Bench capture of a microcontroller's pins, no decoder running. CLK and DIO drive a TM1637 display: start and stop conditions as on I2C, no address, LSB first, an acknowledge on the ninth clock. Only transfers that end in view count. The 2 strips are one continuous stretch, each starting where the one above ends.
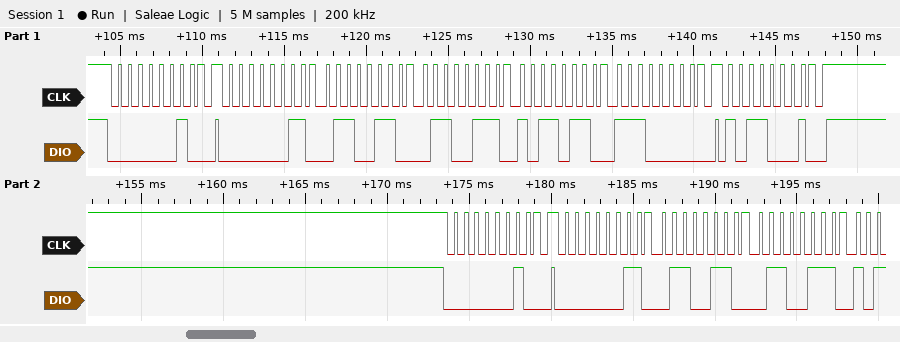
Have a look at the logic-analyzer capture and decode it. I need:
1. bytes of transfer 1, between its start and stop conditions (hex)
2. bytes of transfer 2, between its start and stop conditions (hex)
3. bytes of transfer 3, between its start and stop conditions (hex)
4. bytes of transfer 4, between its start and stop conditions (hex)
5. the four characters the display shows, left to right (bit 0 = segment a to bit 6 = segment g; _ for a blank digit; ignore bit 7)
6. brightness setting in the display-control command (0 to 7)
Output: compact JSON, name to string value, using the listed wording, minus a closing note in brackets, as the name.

{"bytes of transfer 1, between its start and stop conditions": "40", "bytes of transfer 2, between its start and stop conditions": "C0 66 E6 6D 07", "bytes of transfer 3, between its start and stop conditions": "8D", "bytes of transfer 4, between its start and stop conditions": "40", "the four characters the display shows, left to right": "4457", "brightness setting in the display-control command": "5"}
